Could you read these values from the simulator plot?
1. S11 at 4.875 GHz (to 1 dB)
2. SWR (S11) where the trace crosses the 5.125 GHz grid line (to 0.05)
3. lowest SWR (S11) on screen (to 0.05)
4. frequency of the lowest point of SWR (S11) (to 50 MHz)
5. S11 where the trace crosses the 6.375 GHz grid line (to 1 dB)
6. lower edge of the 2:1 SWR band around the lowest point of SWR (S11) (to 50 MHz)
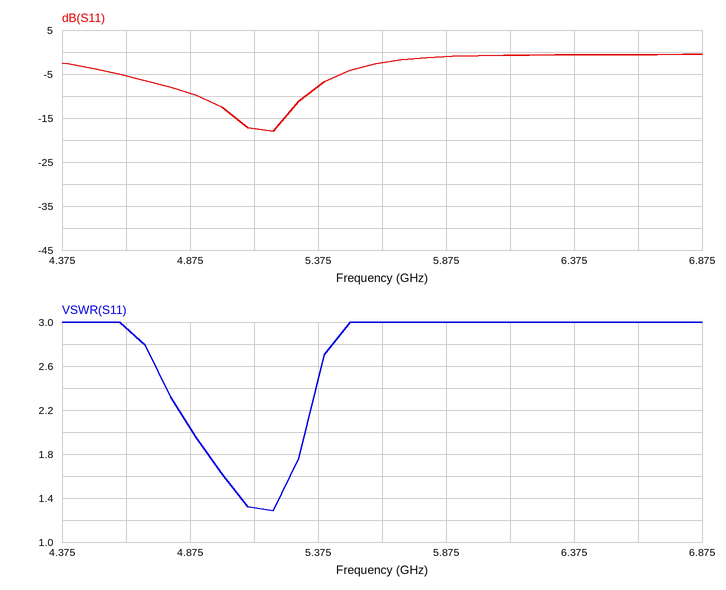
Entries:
-9 dB
1.30
1.30
5.20 GHz
-1 dB
4.90 GHz
